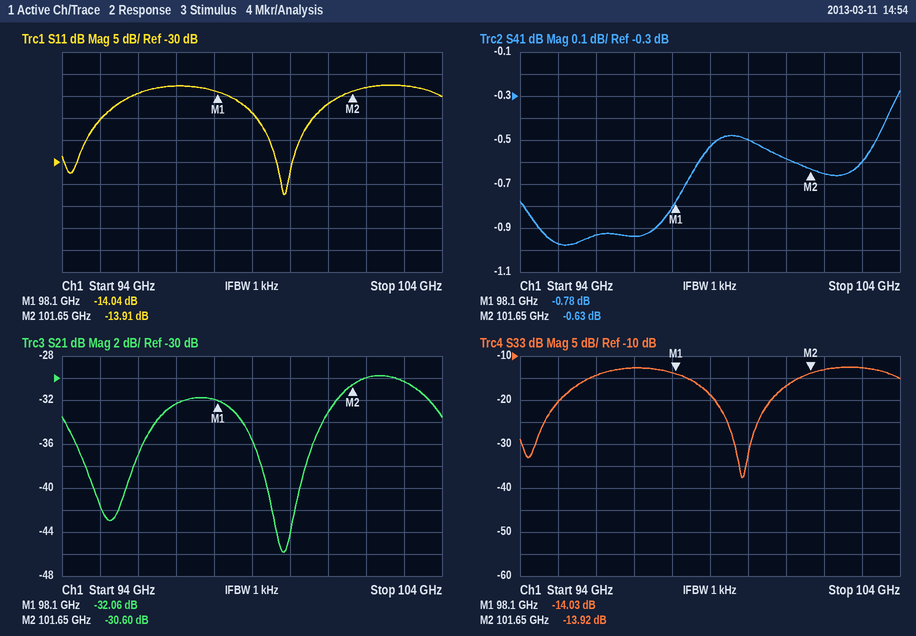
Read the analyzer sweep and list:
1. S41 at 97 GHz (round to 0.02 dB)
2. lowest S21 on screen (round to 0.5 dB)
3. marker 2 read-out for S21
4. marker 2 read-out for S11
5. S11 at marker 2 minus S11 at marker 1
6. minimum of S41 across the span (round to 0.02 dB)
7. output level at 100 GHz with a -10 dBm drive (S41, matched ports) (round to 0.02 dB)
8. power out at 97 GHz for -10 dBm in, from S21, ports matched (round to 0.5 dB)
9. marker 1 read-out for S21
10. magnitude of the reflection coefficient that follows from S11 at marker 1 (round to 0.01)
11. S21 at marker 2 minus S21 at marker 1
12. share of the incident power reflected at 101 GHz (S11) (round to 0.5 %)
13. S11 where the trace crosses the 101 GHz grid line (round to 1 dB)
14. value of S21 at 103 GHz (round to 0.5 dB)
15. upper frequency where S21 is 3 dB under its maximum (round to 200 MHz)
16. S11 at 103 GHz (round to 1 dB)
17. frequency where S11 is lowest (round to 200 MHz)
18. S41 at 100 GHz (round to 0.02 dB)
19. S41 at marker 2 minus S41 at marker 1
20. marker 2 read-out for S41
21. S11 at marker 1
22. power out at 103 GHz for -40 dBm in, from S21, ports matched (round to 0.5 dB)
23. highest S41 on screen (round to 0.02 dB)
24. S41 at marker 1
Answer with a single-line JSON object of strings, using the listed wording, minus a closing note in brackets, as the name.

{"S41 at 97 GHz": "-0.94 dB", "lowest S21 on screen": "-46.0 dB", "marker 2 read-out for S21": "-30.60 dB", "marker 2 read-out for S11": "-13.91 dB", "S11 at marker 2 minus S11 at marker 1": "0.13 dB", "minimum of S41 across the span": "-0.98 dB", "output level at 100 GHz with a -10 dBm drive (S41, matched ports)": "-10.50 dBm", "power out at 97 GHz for -10 dBm in, from S21, ports matched": "-42.5 dBm", "marker 1 read-out for S21": "-32.06 dB", "magnitude of the reflection coefficient that follows from S11 at marker 1": "0.20", "S21 at marker 2 minus S21 at marker 1": "1.46 dB", "share of the incident power reflected at 101 GHz (S11)": "2.0 %", "S11 where the trace crosses the 101 GHz grid line": "-17 dB", "value of S21 at 103 GHz": "-30.5 dB", "upper frequency where S21 is 3 dB under its maximum": "103.8 GHz", "S11 at 103 GHz": "-13 dB", "frequency where S11 is lowest": "99.8 GHz", "S41 at 100 GHz": "-0.50 dB", "S41 at marker 2 minus S41 at marker 1": "0.15 dB", "marker 2 read-out for S41": "-0.63 dB", "S11 at marker 1": "-14.04 dB", "power out at 103 GHz for -40 dBm in, from S21, ports matched": "-70.5 dBm", "highest S41 on screen": "-0.28 dB", "S41 at marker 1": "-0.78 dB"}
